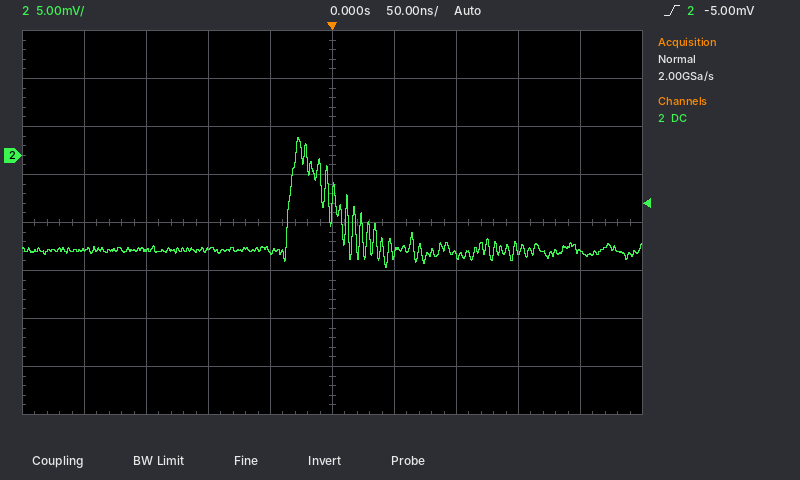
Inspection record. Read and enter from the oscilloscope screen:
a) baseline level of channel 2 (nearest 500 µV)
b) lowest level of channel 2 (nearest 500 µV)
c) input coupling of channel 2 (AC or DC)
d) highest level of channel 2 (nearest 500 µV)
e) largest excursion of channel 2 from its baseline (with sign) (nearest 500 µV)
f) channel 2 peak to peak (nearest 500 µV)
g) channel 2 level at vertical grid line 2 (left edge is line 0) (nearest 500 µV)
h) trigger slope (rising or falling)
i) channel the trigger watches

-10.0 mV
-11.5 mV
DC
2.0 mV
+12.0 mV
13.5 mV
-10.0 mV
rising
channel 2
